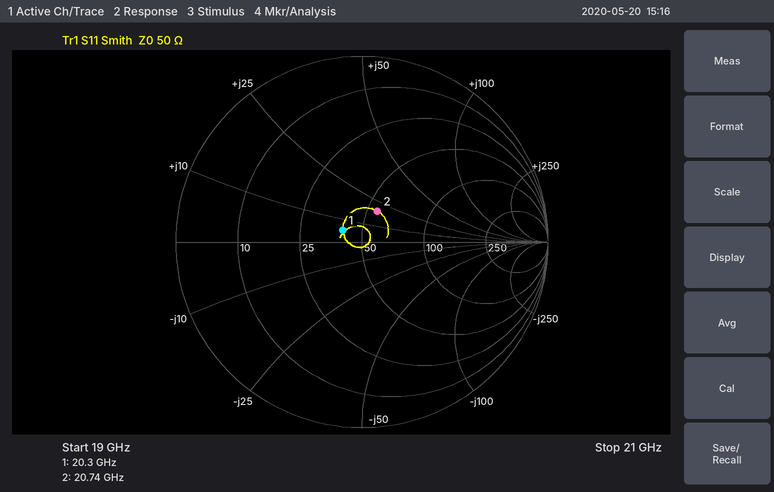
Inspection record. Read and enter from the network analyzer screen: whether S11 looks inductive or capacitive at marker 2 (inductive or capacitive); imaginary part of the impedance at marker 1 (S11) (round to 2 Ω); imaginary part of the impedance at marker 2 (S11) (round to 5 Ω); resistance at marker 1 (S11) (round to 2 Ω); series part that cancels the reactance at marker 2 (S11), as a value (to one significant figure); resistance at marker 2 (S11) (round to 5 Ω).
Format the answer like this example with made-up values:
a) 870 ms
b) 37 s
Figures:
a) inductive
b) +6 Ω
c) +20 Ω
d) 40 Ω
e) 400 fF
f) 55 Ω
